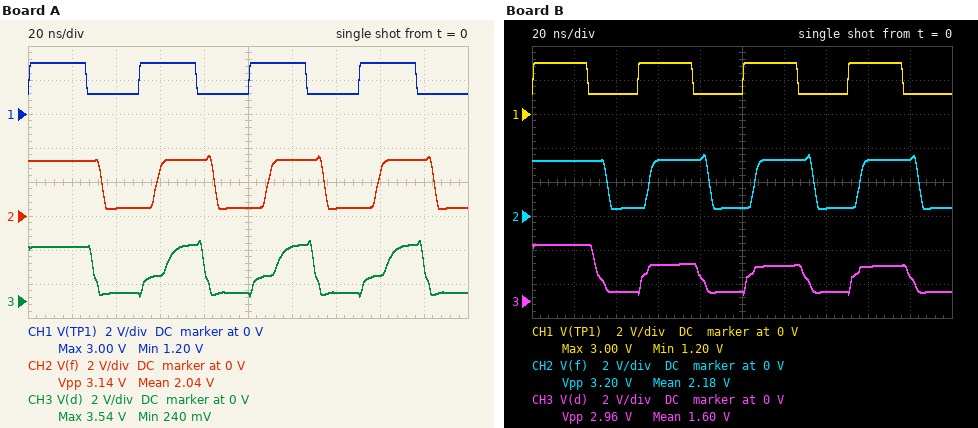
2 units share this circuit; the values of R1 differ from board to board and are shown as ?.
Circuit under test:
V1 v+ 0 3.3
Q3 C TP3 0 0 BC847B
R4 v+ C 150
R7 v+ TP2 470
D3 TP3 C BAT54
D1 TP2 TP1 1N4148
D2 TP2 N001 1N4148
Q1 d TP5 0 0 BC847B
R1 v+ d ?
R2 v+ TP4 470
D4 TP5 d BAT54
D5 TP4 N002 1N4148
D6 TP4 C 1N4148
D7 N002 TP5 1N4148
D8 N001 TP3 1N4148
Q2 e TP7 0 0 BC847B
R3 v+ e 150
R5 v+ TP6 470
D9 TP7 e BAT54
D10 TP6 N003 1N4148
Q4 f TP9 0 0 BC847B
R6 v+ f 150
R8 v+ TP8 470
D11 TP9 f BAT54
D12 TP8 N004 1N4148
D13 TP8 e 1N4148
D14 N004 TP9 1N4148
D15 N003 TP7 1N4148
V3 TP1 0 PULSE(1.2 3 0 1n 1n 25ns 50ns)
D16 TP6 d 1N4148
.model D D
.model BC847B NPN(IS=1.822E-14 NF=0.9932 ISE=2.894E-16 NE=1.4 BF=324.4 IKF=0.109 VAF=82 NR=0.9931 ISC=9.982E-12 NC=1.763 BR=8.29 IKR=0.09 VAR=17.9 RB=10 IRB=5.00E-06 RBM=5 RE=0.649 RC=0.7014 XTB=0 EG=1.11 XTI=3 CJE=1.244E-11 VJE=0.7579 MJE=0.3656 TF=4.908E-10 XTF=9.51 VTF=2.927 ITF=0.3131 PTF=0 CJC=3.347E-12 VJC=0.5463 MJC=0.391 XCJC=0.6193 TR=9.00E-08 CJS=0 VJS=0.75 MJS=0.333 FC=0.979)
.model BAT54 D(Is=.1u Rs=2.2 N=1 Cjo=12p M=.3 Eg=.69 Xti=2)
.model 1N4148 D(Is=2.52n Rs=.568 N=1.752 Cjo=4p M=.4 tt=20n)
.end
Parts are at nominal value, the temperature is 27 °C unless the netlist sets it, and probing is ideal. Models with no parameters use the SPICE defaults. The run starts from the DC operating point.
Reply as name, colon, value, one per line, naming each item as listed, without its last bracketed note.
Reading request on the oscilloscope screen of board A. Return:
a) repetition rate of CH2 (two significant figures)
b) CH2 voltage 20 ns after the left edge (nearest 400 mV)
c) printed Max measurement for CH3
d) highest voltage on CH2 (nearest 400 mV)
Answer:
repetition rate of CH2: 20 MHz
CH2 voltage 20 ns after the left edge: 3.2 V
printed Max measurement for CH3: 3.54 V
highest voltage on CH2: 3.6 V
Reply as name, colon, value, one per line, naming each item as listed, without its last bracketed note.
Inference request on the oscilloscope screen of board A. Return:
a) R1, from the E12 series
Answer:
R1, from the E12 series: 270 Ω
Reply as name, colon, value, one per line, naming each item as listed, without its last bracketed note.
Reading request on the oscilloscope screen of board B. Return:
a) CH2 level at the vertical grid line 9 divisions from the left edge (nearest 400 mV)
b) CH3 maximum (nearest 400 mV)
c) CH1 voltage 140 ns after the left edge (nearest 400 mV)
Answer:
CH2 level at the vertical grid line 9 divisions from the left edge: 3.2 V
CH3 maximum: 3.2 V
CH1 voltage 140 ns after the left edge: 1.2 V
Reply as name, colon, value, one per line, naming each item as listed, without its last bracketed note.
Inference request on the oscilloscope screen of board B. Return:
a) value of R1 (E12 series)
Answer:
value of R1: 47 Ω
